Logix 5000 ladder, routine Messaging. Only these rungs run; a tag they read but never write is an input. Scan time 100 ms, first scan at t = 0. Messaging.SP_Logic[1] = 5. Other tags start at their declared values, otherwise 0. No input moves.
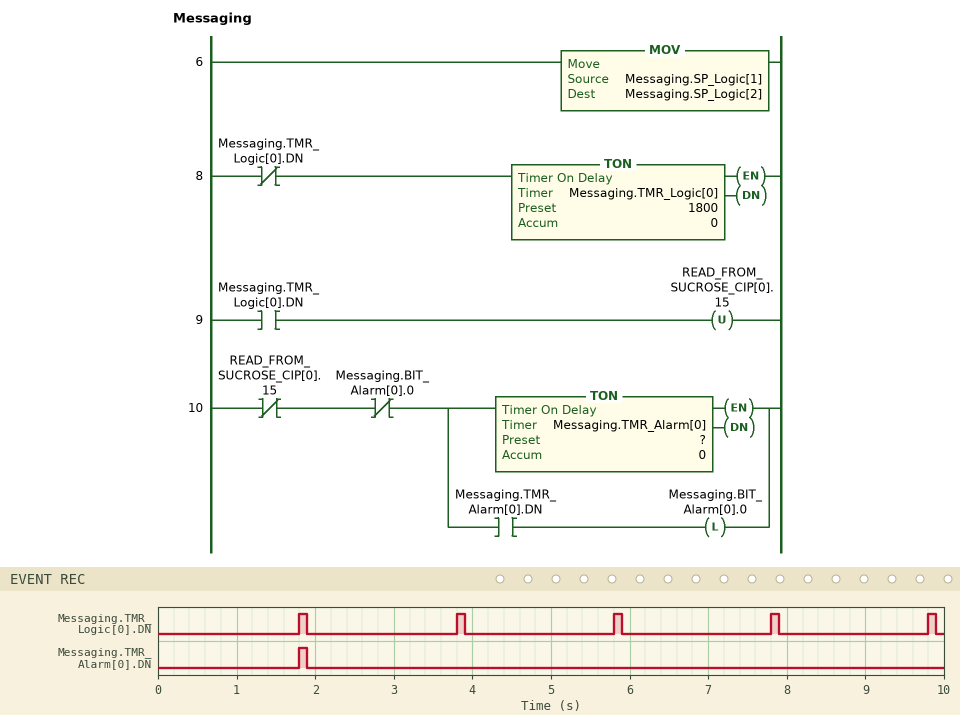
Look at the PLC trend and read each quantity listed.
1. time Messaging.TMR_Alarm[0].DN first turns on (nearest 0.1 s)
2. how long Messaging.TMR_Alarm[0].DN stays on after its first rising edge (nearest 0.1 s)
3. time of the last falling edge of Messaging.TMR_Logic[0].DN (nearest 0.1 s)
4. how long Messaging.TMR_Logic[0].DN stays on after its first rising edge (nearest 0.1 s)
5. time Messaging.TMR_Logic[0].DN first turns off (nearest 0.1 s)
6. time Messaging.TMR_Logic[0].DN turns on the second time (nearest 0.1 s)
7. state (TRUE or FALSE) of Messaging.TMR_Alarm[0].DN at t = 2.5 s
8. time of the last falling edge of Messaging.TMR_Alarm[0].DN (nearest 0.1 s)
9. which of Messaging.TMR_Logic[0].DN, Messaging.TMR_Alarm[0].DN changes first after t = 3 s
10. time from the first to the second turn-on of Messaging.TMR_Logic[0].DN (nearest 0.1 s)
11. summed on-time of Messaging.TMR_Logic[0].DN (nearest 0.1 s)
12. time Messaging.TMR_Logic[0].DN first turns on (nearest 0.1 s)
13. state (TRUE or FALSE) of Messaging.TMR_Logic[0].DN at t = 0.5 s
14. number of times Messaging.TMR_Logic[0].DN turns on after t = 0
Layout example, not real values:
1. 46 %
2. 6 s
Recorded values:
1. 1.8 s
2. 0.1 s
3. 9.9 s
4. 0.1 s
5. 1.9 s
6. 3.8 s
7. FALSE
8. 1.9 s
9. Messaging.TMR_Logic[0].DN
10. 2.0 s
11. 0.5 s
12. 1.8 s
13. FALSE
14. 5
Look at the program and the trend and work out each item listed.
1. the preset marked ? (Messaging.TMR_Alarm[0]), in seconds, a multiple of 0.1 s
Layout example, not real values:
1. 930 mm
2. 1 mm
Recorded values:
1. 1.8 s
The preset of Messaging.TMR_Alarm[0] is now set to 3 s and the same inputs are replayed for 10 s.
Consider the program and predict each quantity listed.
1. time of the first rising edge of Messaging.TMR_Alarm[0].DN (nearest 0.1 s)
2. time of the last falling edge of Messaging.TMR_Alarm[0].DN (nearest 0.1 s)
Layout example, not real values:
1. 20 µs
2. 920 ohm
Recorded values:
1. 3.0 s
2. 3.1 s
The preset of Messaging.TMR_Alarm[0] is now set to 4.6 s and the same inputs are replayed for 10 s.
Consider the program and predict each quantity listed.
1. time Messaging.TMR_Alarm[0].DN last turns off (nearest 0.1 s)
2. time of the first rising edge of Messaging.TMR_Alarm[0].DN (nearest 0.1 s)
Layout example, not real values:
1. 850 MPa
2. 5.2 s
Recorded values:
1. 4.7 s
2. 4.6 s
